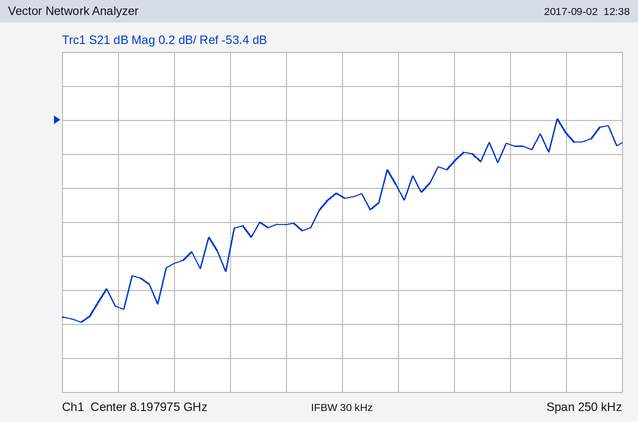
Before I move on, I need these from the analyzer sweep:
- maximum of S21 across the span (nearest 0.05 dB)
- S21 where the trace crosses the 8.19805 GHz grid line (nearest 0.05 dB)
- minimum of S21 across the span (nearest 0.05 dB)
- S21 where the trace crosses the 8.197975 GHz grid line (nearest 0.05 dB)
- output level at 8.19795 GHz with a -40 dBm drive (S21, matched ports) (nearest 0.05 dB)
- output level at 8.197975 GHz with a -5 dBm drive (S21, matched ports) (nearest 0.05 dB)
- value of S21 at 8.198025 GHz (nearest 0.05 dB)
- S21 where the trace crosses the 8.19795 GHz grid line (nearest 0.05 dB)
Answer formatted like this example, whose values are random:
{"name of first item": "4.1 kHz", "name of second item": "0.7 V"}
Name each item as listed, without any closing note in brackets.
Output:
{"maximum of S21 across the span": "-53.40 dB", "S21 where the trace crosses the 8.19805 GHz grid line": "-53.55 dB", "minimum of S21 across the span": "-54.60 dB", "S21 where the trace crosses the 8.197975 GHz grid line": "-53.85 dB", "output level at 8.19795 GHz with a -40 dBm drive (S21, matched ports)": "-94.00 dBm", "output level at 8.197975 GHz with a -5 dBm drive (S21, matched ports)": "-58.85 dBm", "value of S21 at 8.198025 GHz": "-53.65 dB", "S21 where the trace crosses the 8.19795 GHz grid line": "-54.00 dB"}
